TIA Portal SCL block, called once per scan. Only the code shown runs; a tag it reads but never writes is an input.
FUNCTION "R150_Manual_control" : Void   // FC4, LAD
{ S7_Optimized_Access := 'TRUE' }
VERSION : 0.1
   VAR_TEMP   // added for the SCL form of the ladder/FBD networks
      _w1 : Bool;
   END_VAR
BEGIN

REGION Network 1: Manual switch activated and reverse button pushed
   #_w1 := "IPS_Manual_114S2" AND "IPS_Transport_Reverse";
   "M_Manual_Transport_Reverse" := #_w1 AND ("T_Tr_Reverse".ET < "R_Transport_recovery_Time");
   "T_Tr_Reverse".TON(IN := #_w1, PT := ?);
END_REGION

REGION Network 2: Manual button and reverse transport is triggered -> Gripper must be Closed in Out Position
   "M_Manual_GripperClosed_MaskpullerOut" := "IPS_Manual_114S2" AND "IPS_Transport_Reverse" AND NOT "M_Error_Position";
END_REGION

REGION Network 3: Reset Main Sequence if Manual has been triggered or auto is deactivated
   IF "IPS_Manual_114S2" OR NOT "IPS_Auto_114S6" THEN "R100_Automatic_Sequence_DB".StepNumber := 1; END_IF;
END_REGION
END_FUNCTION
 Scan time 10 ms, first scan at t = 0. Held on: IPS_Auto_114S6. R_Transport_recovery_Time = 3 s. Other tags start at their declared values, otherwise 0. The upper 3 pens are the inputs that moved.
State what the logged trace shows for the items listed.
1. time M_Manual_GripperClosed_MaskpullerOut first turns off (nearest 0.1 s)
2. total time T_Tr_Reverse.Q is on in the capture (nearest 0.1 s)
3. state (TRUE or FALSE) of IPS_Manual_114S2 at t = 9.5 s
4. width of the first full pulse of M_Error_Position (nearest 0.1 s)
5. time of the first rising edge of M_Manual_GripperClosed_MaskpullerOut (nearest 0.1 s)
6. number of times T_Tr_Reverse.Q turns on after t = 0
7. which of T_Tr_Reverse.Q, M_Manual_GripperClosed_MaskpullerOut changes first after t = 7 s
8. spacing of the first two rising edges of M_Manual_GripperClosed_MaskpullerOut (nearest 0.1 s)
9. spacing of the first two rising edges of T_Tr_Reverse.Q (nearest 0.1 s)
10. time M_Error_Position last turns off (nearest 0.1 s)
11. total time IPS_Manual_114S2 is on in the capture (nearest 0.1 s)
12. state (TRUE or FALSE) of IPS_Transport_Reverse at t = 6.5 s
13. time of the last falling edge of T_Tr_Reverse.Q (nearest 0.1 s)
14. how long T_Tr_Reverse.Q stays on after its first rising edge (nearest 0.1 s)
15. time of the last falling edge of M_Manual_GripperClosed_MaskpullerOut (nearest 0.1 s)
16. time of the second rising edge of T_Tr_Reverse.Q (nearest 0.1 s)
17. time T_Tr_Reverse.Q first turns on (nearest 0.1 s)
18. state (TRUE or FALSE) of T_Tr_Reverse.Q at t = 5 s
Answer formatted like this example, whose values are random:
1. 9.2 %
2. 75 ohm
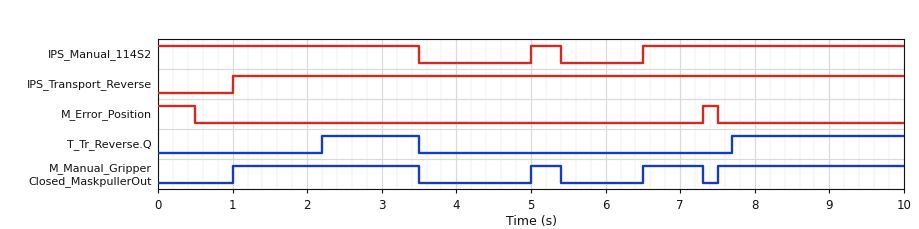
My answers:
1. 3.5 s
2. 3.6 s
3. TRUE
4. 0.2 s
5. 1.0 s
6. 2
7. M_Manual_GripperClosed_MaskpullerOut
8. 4.0 s
9. 5.5 s
10. 7.5 s
11. 7.4 s
12. TRUE
13. 3.5 s
14. 1.3 s
15. 7.3 s
16. 7.7 s
17. 2.2 s
18. FALSE
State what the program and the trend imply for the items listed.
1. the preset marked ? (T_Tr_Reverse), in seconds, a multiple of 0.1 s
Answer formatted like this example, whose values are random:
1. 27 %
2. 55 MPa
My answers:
1. 1.2 s
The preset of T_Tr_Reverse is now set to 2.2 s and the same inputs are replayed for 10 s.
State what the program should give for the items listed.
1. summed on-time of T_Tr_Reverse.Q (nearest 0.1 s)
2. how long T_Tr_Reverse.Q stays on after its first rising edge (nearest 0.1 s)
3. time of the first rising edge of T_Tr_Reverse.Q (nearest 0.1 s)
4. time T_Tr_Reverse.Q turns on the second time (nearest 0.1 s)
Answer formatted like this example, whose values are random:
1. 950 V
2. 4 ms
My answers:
1. 1.6 s
2. 0.3 s
3. 3.2 s
4. 8.7 s
